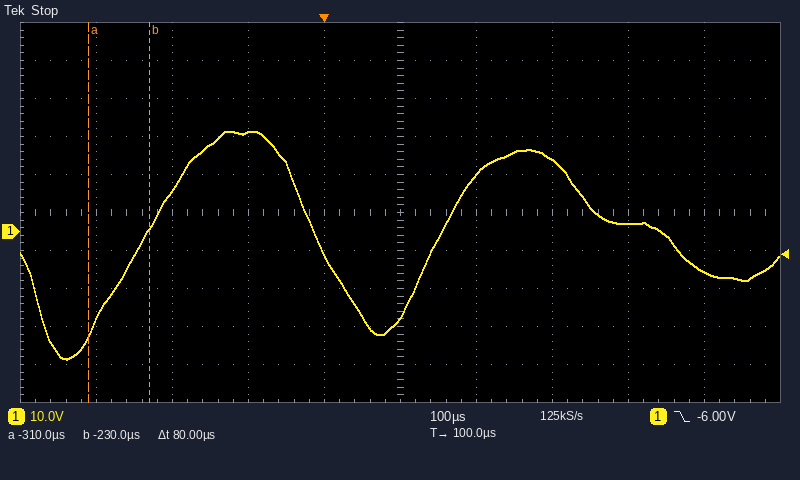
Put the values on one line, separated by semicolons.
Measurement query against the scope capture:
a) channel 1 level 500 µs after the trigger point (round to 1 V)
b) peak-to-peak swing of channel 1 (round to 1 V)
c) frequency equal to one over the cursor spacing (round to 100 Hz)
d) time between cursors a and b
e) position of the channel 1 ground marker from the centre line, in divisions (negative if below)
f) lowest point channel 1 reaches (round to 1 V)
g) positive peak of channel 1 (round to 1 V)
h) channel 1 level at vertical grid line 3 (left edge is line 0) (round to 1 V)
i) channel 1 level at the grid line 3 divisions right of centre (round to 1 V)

-11 V; 60 V; 12.5 kHz; 80 µs; -0.5 div; -34 V; 26 V; 26 V; 2 V
